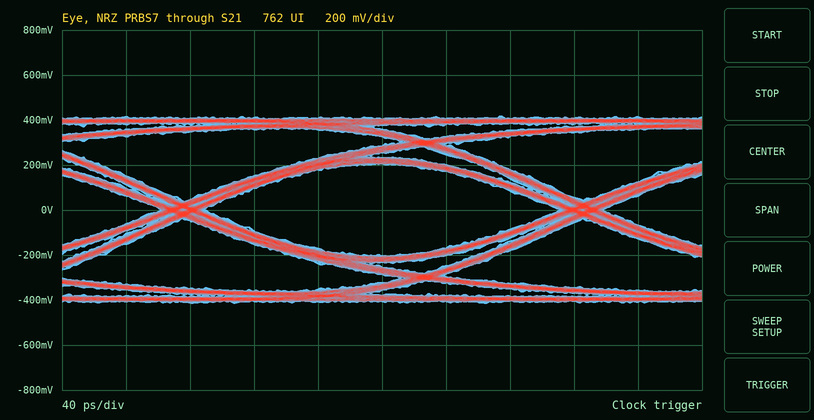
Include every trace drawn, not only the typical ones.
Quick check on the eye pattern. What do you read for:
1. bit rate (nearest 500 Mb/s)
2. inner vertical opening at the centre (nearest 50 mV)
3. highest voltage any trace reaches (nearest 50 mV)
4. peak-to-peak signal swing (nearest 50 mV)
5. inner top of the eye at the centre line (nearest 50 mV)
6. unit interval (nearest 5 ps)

4.0 Gb/s
400 mV
400 mV
850 mV
200 mV
250 ps
